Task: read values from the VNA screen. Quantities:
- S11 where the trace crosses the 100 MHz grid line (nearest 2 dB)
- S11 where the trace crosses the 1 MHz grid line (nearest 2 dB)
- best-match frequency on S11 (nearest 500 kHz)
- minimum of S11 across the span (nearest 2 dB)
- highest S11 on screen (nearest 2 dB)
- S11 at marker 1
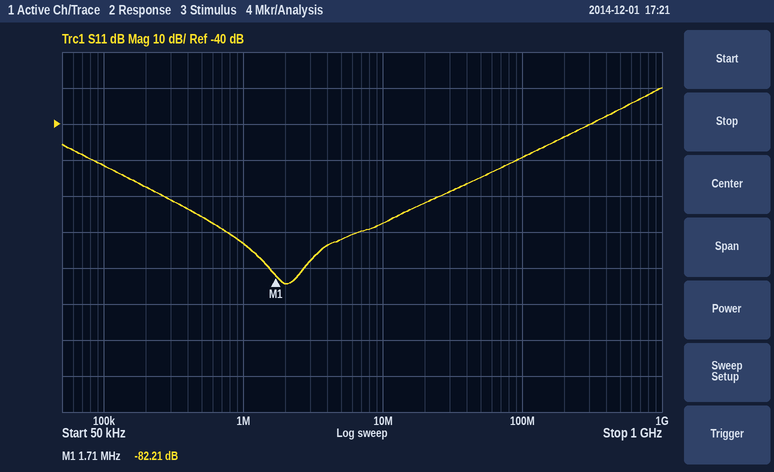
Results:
-50 dB
-74 dB
2.0 MHz
-84 dB
-30 dB
-82.21 dB
